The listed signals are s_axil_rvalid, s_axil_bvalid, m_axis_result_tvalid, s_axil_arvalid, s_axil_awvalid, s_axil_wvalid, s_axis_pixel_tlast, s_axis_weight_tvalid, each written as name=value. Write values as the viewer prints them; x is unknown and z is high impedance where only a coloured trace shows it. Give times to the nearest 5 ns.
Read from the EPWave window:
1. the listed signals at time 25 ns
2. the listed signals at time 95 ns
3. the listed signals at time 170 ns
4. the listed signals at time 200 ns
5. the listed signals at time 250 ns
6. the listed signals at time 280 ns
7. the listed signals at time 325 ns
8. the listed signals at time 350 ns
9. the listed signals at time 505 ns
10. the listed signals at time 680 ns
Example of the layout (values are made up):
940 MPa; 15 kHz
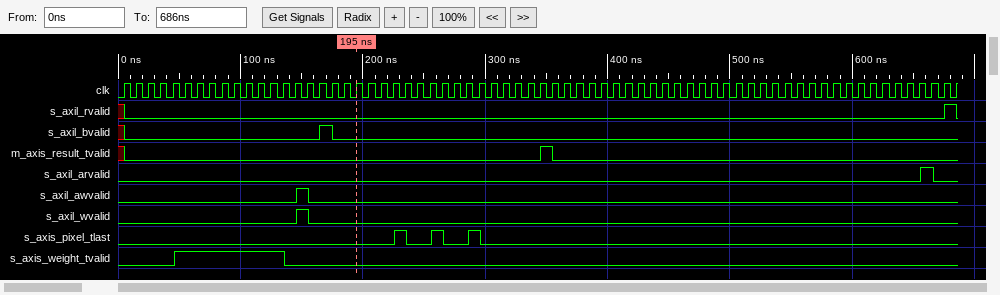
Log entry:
s_axil_rvalid=0, s_axil_bvalid=0, m_axis_result_tvalid=0, s_axil_arvalid=0, s_axil_awvalid=0, s_axil_wvalid=0, s_axis_pixel_tlast=0, s_axis_weight_tvalid=0; s_axil_rvalid=0, s_axil_bvalid=0, m_axis_result_tvalid=0, s_axil_arvalid=0, s_axil_awvalid=0, s_axil_wvalid=0, s_axis_pixel_tlast=0, s_axis_weight_tvalid=1; s_axil_rvalid=0, s_axil_bvalid=1, m_axis_result_tvalid=0, s_axil_arvalid=0, s_axil_awvalid=0, s_axil_wvalid=0, s_axis_pixel_tlast=0, s_axis_weight_tvalid=0; s_axil_rvalid=0, s_axil_bvalid=0, m_axis_result_tvalid=0, s_axil_arvalid=0, s_axil_awvalid=0, s_axil_wvalid=0, s_axis_pixel_tlast=0, s_axis_weight_tvalid=0; s_axil_rvalid=0, s_axil_bvalid=0, m_axis_result_tvalid=0, s_axil_arvalid=0, s_axil_awvalid=0, s_axil_wvalid=0, s_axis_pixel_tlast=0, s_axis_weight_tvalid=0; s_axil_rvalid=0, s_axil_bvalid=0, m_axis_result_tvalid=0, s_axil_arvalid=0, s_axil_awvalid=0, s_axil_wvalid=0, s_axis_pixel_tlast=0, s_axis_weight_tvalid=0; s_axil_rvalid=0, s_axil_bvalid=0, m_axis_result_tvalid=0, s_axil_arvalid=0, s_axil_awvalid=0, s_axil_wvalid=0, s_axis_pixel_tlast=0, s_axis_weight_tvalid=0; s_axil_rvalid=0, s_axil_bvalid=0, m_axis_result_tvalid=1, s_axil_arvalid=0, s_axil_awvalid=0, s_axil_wvalid=0, s_axis_pixel_tlast=0, s_axis_weight_tvalid=0; s_axil_rvalid=0, s_axil_bvalid=0, m_axis_result_tvalid=0, s_axil_arvalid=0, s_axil_awvalid=0, s_axil_wvalid=0, s_axis_pixel_tlast=0, s_axis_weight_tvalid=0; s_axil_rvalid=1, s_axil_bvalid=0, m_axis_result_tvalid=0, s_axil_arvalid=0, s_axil_awvalid=0, s_axil_wvalid=0, s_axis_pixel_tlast=0, s_axis_weight_tvalid=0
